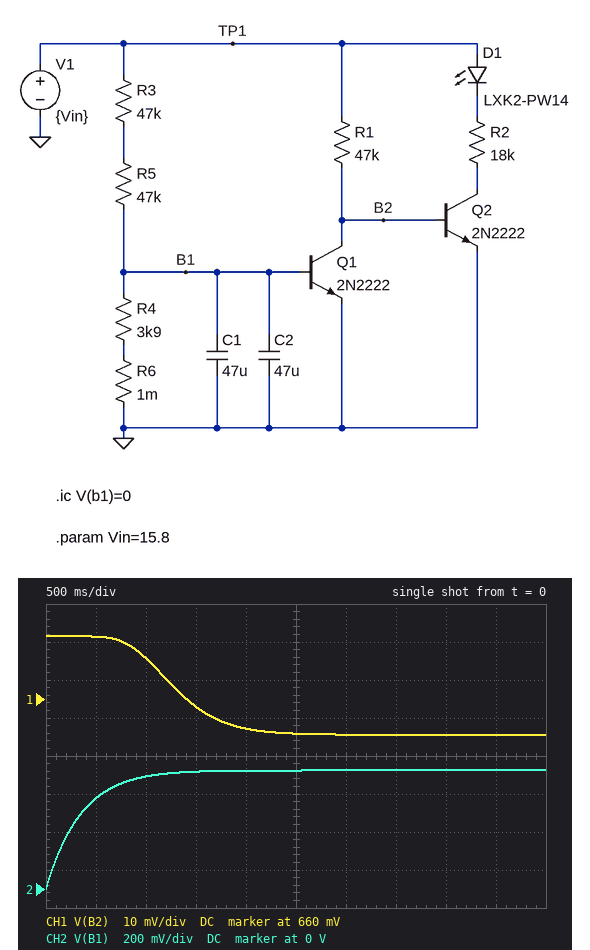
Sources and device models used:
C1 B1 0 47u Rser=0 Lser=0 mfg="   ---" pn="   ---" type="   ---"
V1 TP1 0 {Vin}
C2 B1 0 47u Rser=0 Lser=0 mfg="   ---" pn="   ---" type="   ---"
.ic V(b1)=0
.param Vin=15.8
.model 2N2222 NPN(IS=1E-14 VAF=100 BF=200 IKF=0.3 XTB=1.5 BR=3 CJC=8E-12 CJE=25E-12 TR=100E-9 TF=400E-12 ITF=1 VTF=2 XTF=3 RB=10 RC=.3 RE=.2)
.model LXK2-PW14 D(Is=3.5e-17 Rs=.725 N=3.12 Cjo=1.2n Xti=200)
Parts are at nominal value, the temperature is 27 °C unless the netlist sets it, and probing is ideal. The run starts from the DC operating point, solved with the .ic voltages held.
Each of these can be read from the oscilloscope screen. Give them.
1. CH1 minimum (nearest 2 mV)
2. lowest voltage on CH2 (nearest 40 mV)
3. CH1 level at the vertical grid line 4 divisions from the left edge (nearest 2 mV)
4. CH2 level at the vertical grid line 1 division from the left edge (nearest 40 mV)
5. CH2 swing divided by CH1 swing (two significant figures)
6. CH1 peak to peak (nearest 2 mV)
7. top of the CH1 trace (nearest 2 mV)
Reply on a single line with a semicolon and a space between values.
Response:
650 mV; 0 V; 652 mV; 480 mV; 24; 26 mV; 676 mV
